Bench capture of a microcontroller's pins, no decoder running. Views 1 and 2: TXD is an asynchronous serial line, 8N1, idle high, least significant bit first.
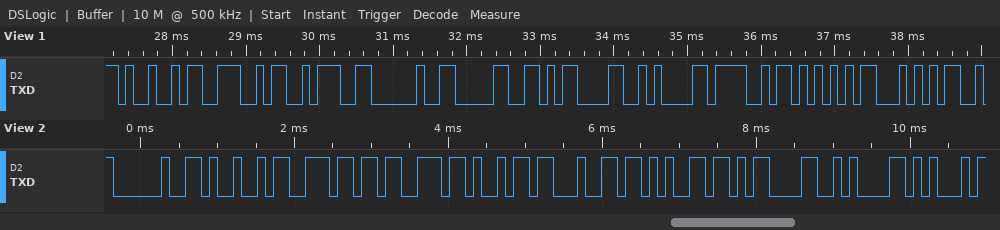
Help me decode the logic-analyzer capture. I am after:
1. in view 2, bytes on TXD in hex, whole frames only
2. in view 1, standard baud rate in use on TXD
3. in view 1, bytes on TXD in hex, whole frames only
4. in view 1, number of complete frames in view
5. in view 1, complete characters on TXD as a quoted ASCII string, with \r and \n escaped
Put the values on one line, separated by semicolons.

20 49 6E 73 69 64 65 0D 0A 45; 9600 baud; 49 4E 3A 20 30 0D 0A 4F 55 54; 10; "IN: 0\r\nOUT"
